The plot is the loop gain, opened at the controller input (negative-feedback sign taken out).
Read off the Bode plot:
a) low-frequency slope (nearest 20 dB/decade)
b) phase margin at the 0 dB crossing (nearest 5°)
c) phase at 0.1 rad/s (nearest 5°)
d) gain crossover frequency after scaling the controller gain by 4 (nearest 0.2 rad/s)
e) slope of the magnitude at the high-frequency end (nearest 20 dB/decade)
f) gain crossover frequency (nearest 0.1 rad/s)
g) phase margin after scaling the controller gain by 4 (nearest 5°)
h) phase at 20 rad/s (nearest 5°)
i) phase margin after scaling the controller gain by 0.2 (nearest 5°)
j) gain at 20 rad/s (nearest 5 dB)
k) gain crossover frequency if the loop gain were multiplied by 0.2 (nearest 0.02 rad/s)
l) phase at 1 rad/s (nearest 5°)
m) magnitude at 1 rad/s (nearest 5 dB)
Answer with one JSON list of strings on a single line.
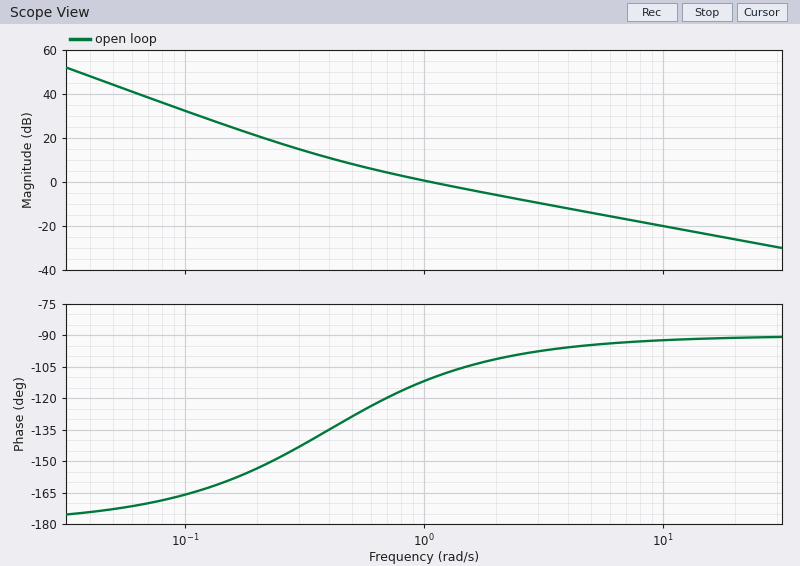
["-40 dB/decade", "70°", "-165°", "4.0 rad/s", "-20 dB/decade", "1.1 rad/s", "85°", "-90°", "40°", "-25 dB", "0.32 rad/s", "-110°", "0 dB"]
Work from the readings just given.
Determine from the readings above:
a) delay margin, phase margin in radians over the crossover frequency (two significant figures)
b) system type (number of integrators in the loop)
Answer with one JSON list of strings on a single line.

["1.1 s", "2"]
